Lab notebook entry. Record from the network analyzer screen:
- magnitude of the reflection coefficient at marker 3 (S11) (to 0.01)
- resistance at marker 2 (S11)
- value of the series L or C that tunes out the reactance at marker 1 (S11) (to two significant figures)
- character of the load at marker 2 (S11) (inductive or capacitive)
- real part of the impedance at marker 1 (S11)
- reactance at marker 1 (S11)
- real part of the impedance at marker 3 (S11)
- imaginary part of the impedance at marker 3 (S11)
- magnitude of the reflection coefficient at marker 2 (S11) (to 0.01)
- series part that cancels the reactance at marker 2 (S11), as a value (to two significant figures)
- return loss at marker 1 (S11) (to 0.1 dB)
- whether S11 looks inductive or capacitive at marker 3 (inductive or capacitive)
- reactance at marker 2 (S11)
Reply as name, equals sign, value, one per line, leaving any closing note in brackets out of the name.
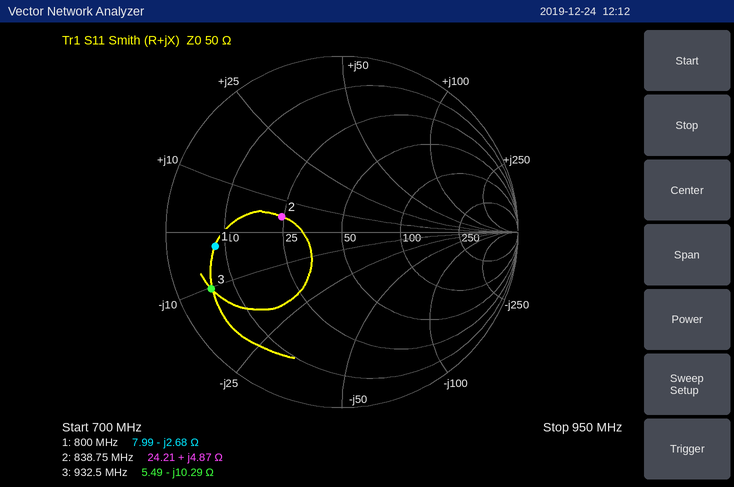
magnitude of the reflection coefficient at marker 3 (S11) = 0.81
resistance at marker 2 = 24.21 Ω
value of the series L or C that tunes out the reactance at marker 1 (S11) = 530 pH
character of the load at marker 2 (S11) = inductive
real part of the impedance at marker 1 = 7.99 Ω
reactance at marker 1 = -2.68 Ω
real part of the impedance at marker 3 = 5.49 Ω
imaginary part of the impedance at marker 3 = -10.29 Ω
magnitude of the reflection coefficient at marker 2 (S11) = 0.35
series part that cancels the reactance at marker 2 (S11), as a value = 39 pF
return loss at marker 1 (S11) = 2.8 dB
whether S11 looks inductive or capacitive at marker 3 = capacitive
reactance at marker 2 = +4.87 Ω
